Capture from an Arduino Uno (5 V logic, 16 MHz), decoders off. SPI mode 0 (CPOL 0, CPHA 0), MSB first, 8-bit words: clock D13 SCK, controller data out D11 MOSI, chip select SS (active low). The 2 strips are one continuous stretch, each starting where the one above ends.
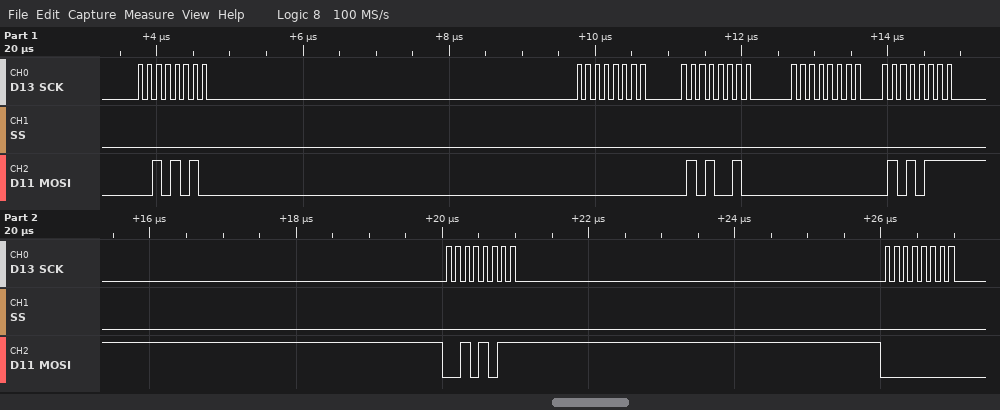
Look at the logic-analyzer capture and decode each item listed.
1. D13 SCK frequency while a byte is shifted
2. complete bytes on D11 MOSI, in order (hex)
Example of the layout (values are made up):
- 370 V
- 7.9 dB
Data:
- 8 MHz
- 2A 00 52 00 57 2B 00
